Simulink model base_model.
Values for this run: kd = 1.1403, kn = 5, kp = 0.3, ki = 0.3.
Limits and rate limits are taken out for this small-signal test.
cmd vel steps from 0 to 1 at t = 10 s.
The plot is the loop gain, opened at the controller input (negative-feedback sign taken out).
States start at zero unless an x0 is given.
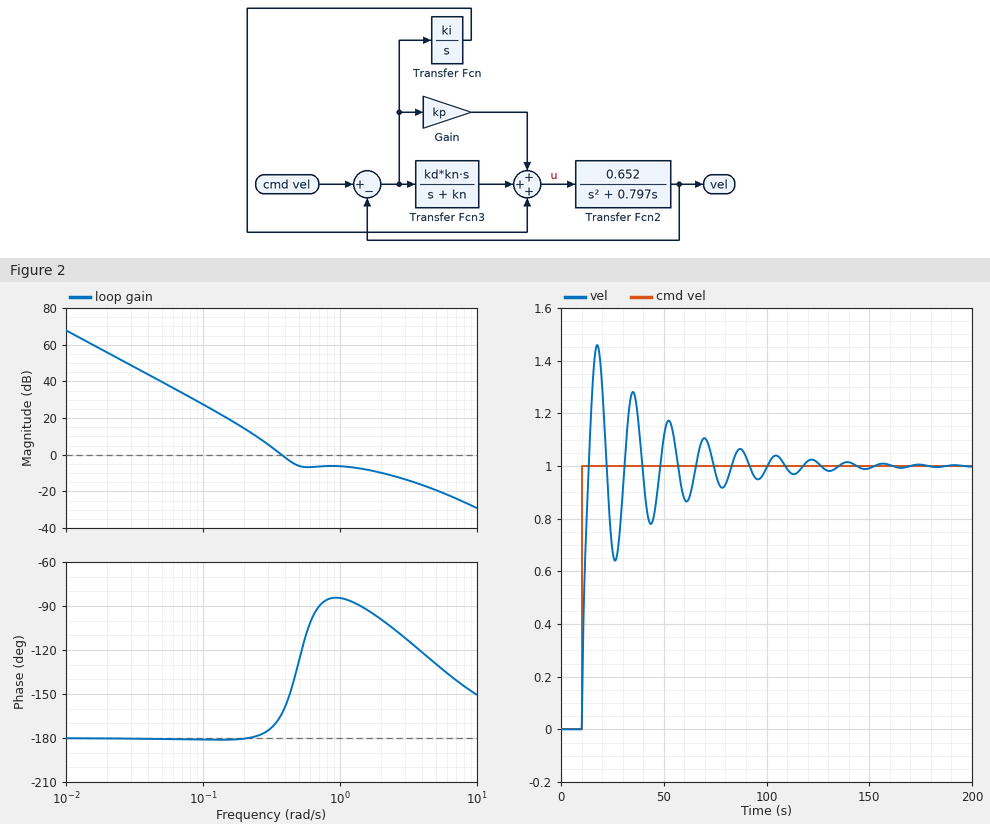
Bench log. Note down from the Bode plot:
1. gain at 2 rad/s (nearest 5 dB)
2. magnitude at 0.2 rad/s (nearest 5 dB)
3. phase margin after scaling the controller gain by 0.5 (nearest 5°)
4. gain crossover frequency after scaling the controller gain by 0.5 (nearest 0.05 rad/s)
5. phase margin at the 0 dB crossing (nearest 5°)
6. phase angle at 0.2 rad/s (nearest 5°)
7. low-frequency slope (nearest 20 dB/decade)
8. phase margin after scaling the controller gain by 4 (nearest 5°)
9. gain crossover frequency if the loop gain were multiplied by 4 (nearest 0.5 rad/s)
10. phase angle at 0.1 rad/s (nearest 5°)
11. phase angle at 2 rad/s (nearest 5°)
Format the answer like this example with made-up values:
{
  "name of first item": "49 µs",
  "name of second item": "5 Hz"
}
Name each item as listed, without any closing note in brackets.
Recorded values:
{
  "gain at 2 rad/s": "-10 dB",
  "magnitude at 0.2 rad/s": "15 dB",
  "phase margin after scaling the controller gain by 0.5": "5°",
  "gain crossover frequency after scaling the controller gain by 0.5": "0.30 rad/s",
  "phase margin at the 0 dB crossing": "15°",
  "phase angle at 0.2 rad/s": "-180°",
  "low-frequency slope": "-40 dB/decade",
  "phase margin after scaling the controller gain by 4": "75°",
  "gain crossover frequency if the loop gain were multiplied by 4": "2.5 rad/s",
  "phase angle at 0.1 rad/s": "-180°",
  "phase angle at 2 rad/s": "-100°"
}
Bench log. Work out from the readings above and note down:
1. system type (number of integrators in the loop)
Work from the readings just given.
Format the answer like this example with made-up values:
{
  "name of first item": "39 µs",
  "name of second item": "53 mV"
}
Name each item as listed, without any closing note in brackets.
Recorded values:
{
  "system type": "2"
}
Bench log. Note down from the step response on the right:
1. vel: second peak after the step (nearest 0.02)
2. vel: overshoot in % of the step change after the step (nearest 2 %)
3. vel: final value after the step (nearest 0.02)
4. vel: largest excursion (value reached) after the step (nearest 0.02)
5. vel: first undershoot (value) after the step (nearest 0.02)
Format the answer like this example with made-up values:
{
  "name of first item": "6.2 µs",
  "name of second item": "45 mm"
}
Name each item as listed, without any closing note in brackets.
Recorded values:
{
  "vel: second peak after the step": "1.28",
  "vel: overshoot in % of the step change after the step": "46 %",
  "vel: final value after the step": "1.00",
  "vel: largest excursion (value reached) after the step": "1.46",
  "vel: first undershoot (value) after the step": "0.64"
}
